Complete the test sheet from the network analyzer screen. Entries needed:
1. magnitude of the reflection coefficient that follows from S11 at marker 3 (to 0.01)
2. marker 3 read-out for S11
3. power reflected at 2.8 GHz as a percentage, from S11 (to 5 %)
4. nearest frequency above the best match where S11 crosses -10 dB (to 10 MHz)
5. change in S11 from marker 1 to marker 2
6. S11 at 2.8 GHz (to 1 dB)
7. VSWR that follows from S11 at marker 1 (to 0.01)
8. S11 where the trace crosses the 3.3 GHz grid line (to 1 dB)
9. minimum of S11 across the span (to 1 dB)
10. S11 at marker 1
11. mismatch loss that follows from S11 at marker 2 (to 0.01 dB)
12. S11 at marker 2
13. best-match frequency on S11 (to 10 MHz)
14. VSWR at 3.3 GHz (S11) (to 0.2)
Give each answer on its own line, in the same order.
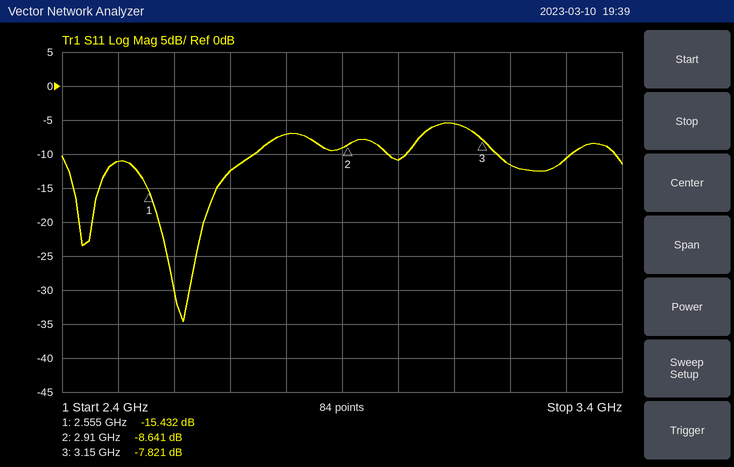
0.41
-7.821 dB
20 %
2.74 GHz
6.791 dB
-7 dB
1.41
-11 dB
-35 dB
-15.432 dB
0.64 dB
-8.641 dB
2.62 GHz
1.8
